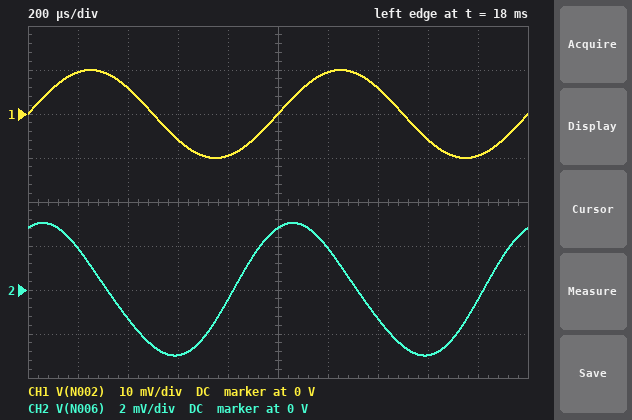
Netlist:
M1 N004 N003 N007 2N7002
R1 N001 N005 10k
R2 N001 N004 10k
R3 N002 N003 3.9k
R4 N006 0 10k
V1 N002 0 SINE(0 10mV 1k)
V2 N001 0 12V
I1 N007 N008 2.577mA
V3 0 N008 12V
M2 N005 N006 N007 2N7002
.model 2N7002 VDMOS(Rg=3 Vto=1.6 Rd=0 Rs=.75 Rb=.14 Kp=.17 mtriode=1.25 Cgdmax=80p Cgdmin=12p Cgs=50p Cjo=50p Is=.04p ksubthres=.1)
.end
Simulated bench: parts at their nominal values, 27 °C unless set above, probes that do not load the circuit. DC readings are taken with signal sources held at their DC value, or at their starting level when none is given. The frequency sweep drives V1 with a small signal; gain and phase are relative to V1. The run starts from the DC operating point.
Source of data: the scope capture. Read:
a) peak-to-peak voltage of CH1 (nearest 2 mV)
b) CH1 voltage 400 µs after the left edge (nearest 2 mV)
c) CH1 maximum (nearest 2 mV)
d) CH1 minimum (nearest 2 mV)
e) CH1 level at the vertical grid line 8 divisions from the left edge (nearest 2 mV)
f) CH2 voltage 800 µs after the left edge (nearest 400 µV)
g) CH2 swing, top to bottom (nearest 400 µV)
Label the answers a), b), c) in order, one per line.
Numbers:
a) 20 mV
b) 6 mV
c) 10 mV
d) -10 mV
e) -6 mV
f) -400 µV
g) 6.0 mV
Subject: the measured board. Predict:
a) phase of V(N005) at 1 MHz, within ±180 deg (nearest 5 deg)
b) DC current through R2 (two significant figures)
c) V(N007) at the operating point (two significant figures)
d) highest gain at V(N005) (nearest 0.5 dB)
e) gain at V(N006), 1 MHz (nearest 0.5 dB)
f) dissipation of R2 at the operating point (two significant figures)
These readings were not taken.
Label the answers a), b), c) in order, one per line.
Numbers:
a) -15 deg
b) 1.3 mA
c) -1.7 V
d) 37.5 dB
e) -7.0 dB
f) 17 mW
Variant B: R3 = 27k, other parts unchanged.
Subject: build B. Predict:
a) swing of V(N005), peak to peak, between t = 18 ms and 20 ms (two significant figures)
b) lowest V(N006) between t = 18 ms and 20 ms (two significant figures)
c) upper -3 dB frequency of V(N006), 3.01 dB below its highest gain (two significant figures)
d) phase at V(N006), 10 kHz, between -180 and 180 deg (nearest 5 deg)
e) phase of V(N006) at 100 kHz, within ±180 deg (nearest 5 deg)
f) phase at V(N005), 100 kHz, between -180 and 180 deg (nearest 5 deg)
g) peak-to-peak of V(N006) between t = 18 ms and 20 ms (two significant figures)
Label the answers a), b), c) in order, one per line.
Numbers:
a) 920 mV
b) -2.1 mV
c) 110 kHz
d) 0 deg
e) -25 deg
f) -90 deg
g) 4.2 mV
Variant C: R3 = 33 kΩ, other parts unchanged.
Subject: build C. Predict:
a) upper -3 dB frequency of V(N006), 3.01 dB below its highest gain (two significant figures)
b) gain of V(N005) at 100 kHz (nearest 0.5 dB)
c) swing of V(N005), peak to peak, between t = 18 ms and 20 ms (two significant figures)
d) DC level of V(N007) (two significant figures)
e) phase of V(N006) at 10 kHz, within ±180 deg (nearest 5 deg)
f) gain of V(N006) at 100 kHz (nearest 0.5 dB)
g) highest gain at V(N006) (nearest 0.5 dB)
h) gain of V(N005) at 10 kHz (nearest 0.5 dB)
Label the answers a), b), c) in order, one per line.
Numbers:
a) 110 kHz
b) -8.0 dB
c) 830 mV
d) -1.7 V
e) 0 deg
f) -15.5 dB
g) -13.0 dB
h) 14.0 dB
